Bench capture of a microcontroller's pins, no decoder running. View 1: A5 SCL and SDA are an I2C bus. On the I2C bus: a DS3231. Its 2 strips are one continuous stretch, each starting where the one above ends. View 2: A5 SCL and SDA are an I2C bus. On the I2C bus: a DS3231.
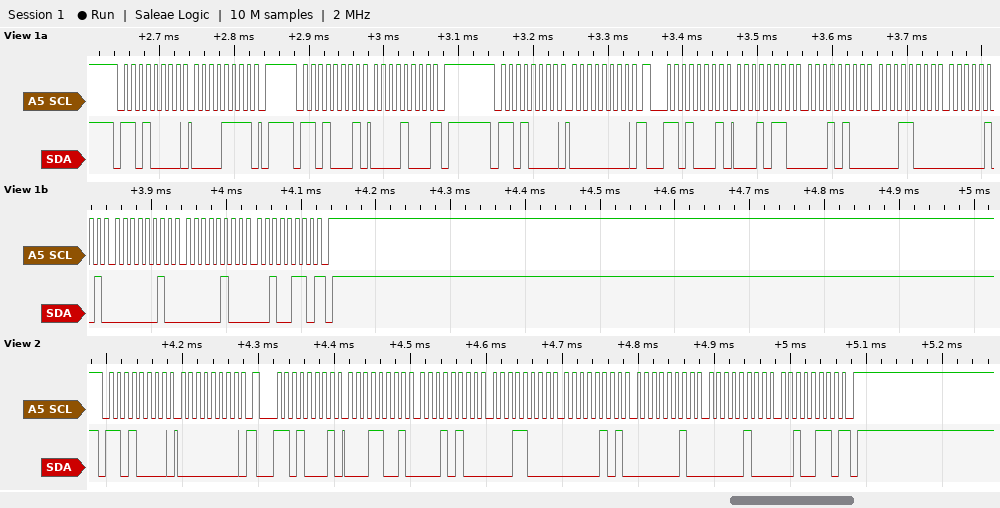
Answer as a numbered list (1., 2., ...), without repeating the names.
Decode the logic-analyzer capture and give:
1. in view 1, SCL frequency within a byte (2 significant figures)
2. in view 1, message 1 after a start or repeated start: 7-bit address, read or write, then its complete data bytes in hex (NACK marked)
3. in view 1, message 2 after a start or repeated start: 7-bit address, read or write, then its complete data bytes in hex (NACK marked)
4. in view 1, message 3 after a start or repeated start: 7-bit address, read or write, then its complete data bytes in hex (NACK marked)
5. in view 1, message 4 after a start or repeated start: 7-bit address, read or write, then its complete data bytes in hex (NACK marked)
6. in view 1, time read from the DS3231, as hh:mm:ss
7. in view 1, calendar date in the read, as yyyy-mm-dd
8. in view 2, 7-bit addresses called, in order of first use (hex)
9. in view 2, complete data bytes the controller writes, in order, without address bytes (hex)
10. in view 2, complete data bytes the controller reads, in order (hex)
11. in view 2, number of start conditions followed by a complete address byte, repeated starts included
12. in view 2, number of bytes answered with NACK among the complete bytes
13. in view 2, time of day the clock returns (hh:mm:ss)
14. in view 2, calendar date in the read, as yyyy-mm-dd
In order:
1. 100 kHz
2. 0x68 write: 0F
3. 0x68 read: 08 NACK
4. 0x68 write: 00
5. 0x68 read: 16 14 18 05 02 04 26 NACK
6. 18:14:16
7. 2026-04-02
8. 0x68
9. 00
10. 19 14 18 05 02 04 26
11. 2
12. 1
13. 18:14:19
14. 2026-04-02
